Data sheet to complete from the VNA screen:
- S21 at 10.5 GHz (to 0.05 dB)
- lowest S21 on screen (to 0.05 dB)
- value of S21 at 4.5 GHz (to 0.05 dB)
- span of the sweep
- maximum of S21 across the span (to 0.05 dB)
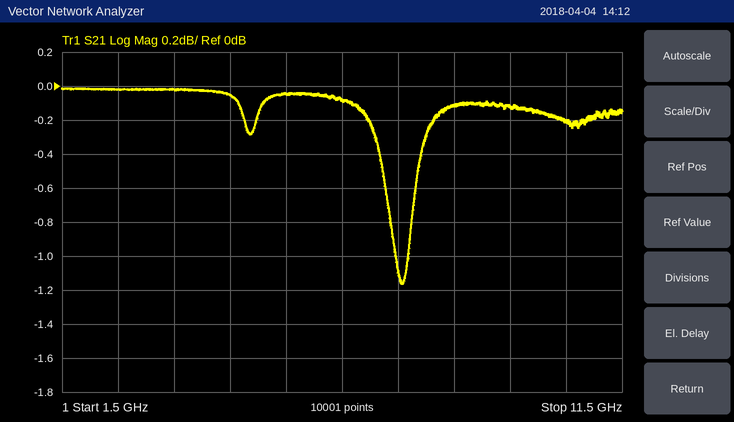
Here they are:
-0.20 dB
-1.15 dB
-0.05 dB
10 GHz
0.00 dB
